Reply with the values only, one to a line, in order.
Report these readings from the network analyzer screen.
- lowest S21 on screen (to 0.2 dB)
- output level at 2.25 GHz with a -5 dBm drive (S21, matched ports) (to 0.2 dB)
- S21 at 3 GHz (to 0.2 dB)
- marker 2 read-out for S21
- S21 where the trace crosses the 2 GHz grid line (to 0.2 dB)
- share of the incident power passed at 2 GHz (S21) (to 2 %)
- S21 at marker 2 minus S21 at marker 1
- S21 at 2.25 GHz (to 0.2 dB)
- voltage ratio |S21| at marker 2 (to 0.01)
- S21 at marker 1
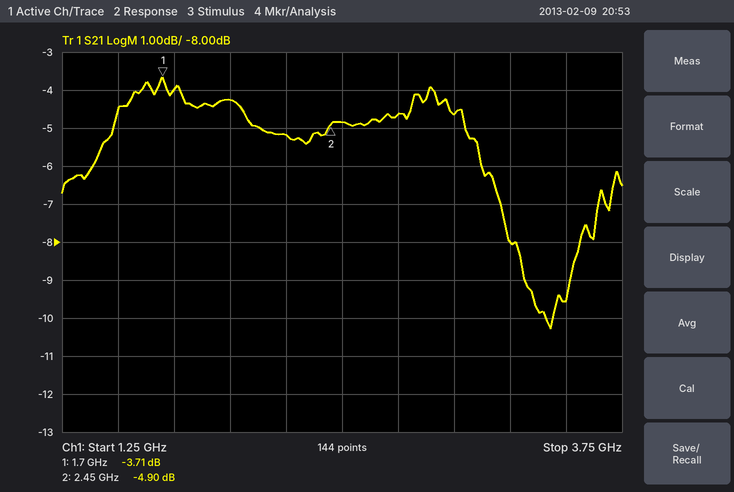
-10.2 dB
-10.2 dBm
-4.6 dB
-4.90 dB
-4.2 dB
38 %
-1.19 dB
-5.2 dB
0.57
-3.71 dB
